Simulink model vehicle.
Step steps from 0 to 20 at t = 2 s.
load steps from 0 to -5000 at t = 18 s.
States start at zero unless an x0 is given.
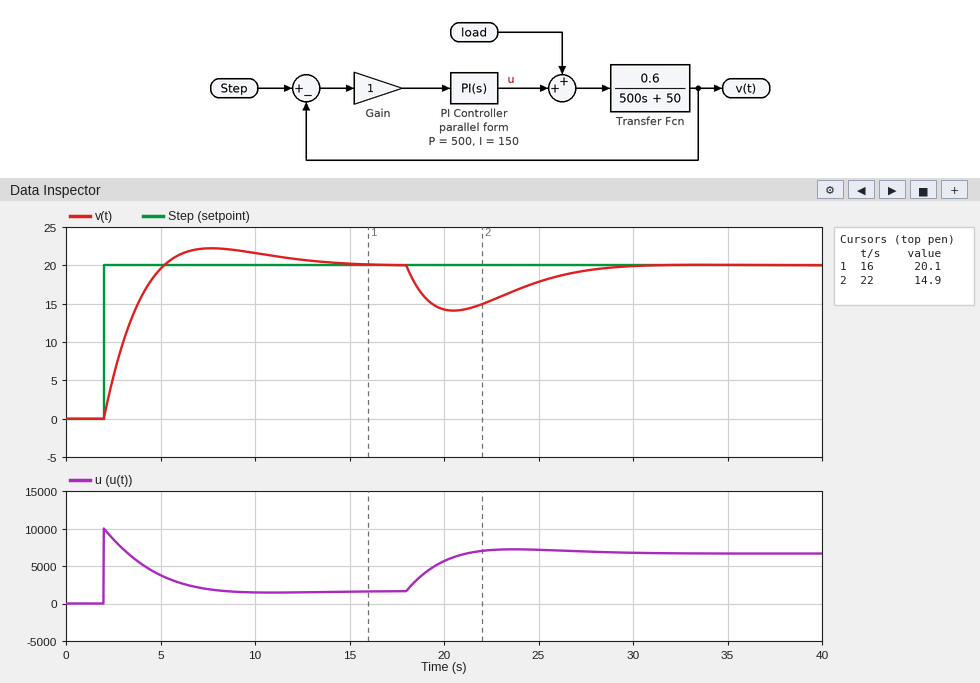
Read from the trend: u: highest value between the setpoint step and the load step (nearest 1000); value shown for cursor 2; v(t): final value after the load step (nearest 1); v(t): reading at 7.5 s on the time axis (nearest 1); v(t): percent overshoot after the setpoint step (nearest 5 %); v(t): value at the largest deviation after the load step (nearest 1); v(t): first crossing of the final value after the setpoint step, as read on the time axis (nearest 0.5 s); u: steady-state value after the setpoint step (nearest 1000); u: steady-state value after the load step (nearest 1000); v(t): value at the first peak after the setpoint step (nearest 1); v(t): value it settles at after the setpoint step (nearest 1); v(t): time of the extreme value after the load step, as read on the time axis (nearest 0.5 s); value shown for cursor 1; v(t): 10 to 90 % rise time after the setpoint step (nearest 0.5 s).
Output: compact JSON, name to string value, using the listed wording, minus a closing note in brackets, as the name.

{"u: highest value between the setpoint step and the load step": "10000", "value shown for cursor 2": "14.9", "v(t): final value after the load step": "20", "v(t): reading at 7.5 s on the time axis": "22", "v(t): percent overshoot after the setpoint step": "10 %", "v(t): value at the largest deviation after the load step": "14", "v(t): first crossing of the final value after the setpoint step, as read on the time axis": "5.0 s", "u: steady-state value after the setpoint step": "2000", "u: steady-state value after the load step": "7000", "v(t): value at the first peak after the setpoint step": "22", "v(t): value it settles at after the setpoint step": "20", "v(t): time of the extreme value after the load step, as read on the time axis": "20.5 s", "value shown for cursor 1": "20.1", "v(t): 10 to 90 % rise time after the setpoint step": "2.5 s"}
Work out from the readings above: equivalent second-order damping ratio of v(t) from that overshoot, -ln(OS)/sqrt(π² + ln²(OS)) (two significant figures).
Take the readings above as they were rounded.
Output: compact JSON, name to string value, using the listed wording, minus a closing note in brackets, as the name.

{"equivalent second-order damping ratio of v(t) from that overshoot, -ln(OS)/sqrt(π² + ln²(OS))": "0.59"}
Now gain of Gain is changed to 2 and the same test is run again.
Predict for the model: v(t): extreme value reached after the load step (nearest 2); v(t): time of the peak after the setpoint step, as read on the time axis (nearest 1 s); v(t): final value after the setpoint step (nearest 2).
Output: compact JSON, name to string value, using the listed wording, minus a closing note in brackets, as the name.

{"v(t): extreme value reached after the load step": "16", "v(t): time of the peak after the setpoint step, as read on the time axis": "6 s", "v(t): final value after the setpoint step": "20"}
